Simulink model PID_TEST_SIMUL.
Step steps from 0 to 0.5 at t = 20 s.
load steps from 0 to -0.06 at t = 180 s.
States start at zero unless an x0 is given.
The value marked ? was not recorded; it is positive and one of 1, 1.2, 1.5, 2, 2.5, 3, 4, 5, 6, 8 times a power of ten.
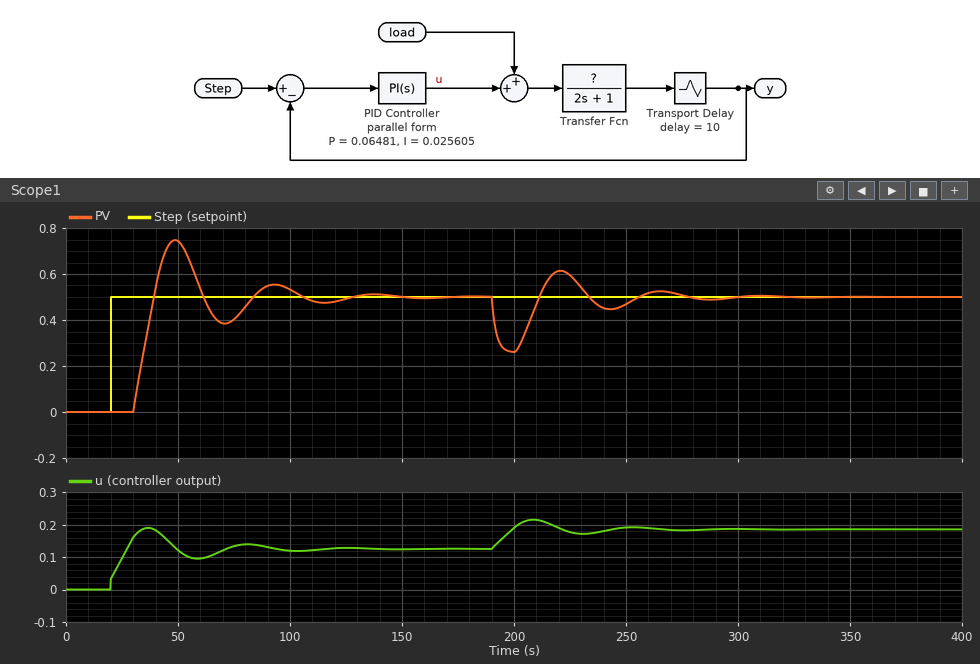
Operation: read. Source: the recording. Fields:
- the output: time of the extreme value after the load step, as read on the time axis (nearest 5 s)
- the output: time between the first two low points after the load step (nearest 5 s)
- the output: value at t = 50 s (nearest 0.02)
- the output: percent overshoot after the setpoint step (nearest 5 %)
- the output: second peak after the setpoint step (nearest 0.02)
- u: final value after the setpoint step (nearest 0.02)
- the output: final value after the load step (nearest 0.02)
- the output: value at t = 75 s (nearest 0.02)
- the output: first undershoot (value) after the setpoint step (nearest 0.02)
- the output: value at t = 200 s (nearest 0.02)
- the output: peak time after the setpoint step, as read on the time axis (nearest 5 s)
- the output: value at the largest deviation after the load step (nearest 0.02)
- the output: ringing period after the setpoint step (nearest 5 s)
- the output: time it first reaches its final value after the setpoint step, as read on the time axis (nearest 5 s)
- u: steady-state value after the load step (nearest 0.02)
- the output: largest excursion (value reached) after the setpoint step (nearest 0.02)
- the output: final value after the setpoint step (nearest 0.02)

200 s
45 s
0.74
50 %
0.56
0.12
0.50
0.40
0.38
0.26
50 s
0.26
45 s
40 s
0.18
0.74
0.50
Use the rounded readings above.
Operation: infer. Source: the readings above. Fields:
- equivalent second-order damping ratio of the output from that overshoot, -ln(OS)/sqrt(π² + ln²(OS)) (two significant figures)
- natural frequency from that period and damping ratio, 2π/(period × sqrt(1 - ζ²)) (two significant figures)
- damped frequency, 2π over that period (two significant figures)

0.22
0.14 rad/s
0.14 rad/s
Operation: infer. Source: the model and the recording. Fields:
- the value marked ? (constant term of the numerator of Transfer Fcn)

4
